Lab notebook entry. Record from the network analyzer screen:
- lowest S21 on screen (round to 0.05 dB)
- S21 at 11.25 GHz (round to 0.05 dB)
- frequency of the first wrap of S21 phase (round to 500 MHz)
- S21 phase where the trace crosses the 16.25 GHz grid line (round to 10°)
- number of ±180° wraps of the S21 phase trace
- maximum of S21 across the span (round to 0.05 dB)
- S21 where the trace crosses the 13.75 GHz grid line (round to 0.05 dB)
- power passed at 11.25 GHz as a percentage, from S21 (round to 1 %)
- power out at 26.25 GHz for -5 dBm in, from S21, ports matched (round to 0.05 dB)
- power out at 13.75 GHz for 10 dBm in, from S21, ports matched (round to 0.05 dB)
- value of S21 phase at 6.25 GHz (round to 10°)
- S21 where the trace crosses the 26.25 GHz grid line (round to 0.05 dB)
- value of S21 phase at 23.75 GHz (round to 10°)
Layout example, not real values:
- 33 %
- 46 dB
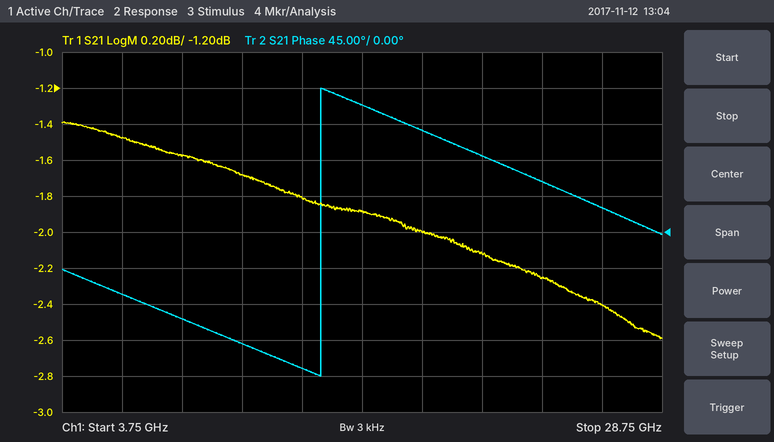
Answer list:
- -2.60 dB
- -1.70 dB
- 14.5 GHz
- 160°
- 1
- -1.40 dB
- -1.80 dB
- 68 %
- -7.40 dBm
- 8.20 dBm
- -80°
- -2.40 dB
- 60°
